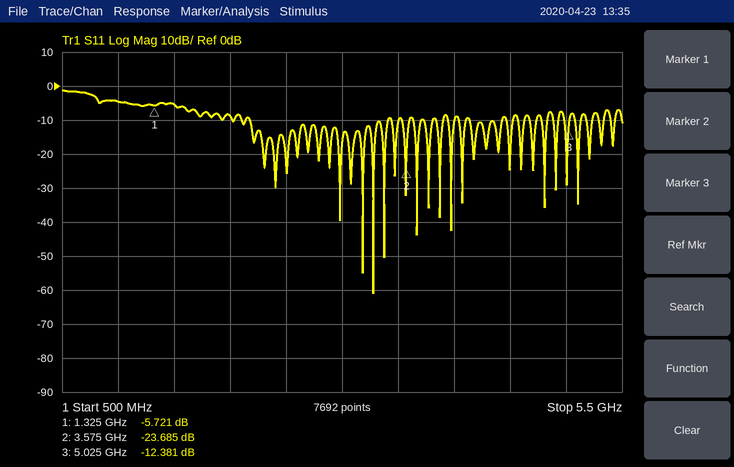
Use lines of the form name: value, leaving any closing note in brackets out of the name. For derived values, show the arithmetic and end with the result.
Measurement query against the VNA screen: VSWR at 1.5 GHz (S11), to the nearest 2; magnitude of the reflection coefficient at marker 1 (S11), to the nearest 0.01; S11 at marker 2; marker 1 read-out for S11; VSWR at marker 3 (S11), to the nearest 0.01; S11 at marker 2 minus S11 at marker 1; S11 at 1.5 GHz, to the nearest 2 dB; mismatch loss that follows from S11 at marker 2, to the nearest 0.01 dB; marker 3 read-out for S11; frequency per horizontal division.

VSWR at 1.5 GHz (S11), to the nearest 2: |Γ| = 10^(-6/20) = 0.5012; VSWR = (1 + 0.5012)/(1 − 0.5012) ≈ 3.01, so 4 to the nearest 2
magnitude of the reflection coefficient at marker 1 (S11), to the nearest 0.01: 10^(-5.721/20) ≈ 0.52
S11 at marker 2: -23.685 dB
marker 1 read-out for S11: -5.721 dB
VSWR at marker 3 (S11), to the nearest 0.01: (1 + 0.2404)/(1 − 0.2404) ≈ 1.63
S11 at marker 2 minus S11 at marker 1: -23.685 − (-5.721) = -17.964 dB
S11 at 1.5 GHz, to the nearest 2 dB: -6 dB
mismatch loss that follows from S11 at marker 2, to the nearest 0.01 dB: −10 log10(1 − 10^(-23.685/10)) ≈ 0.02 dB
marker 3 read-out for S11: -12.381 dB
frequency per horizontal division: 500 MHz
